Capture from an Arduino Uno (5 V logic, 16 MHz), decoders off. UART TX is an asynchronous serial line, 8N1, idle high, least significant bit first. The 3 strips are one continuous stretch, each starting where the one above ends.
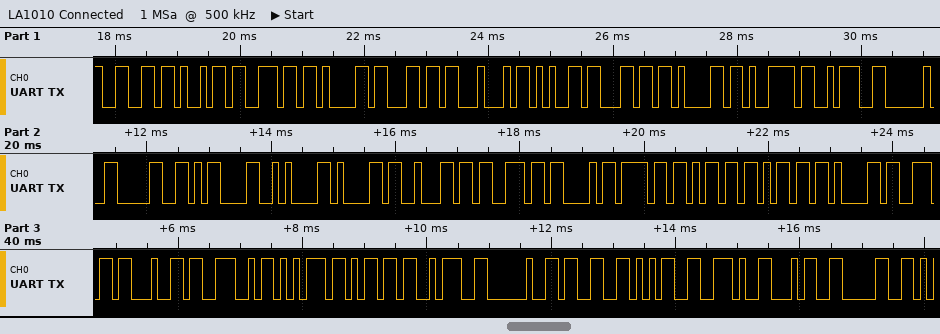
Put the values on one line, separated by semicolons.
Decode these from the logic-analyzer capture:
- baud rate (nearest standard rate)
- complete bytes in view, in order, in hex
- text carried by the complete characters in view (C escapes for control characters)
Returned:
9600 baud; 66 69 6E 61 6C 44 65 6C 61 79 3A 20 30 0D 0A 61 62 73 43 6F 6D 6D 61 6E 64 4E 75 6D 3A 20 33 35 2E 34 30; "finalDelay: 0\r\nabsCommandNum: 35.40"
